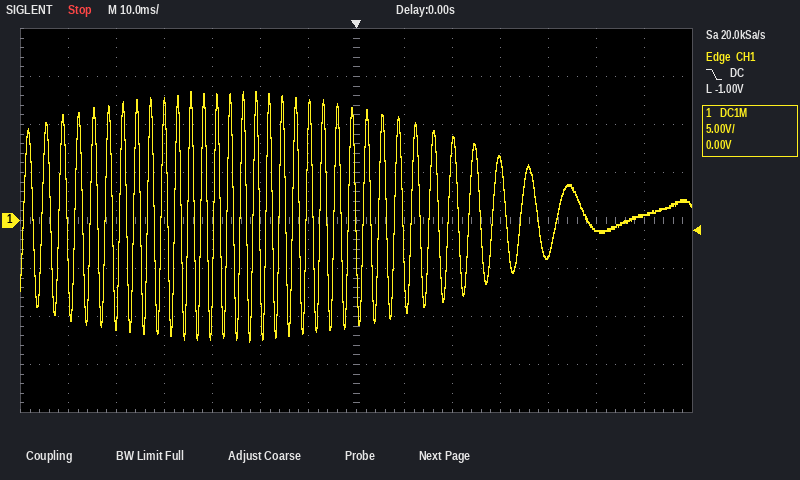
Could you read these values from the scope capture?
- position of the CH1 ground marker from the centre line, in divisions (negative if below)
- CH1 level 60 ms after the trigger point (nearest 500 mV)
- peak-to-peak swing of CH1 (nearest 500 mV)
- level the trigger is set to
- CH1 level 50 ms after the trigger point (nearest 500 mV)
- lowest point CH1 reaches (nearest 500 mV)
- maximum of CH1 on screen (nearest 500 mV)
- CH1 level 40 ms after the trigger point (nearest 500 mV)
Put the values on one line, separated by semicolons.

0.0 div; 500 mV; 26.0 V; -1.00 V; -1.0 V; -12.5 V; 13.5 V; -3.5 V
